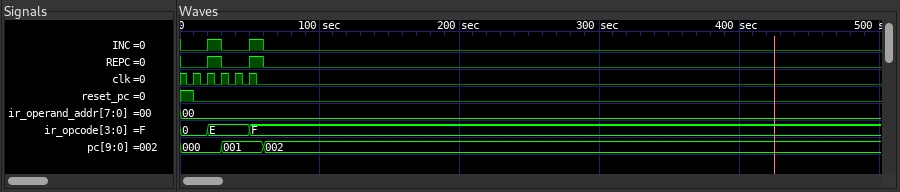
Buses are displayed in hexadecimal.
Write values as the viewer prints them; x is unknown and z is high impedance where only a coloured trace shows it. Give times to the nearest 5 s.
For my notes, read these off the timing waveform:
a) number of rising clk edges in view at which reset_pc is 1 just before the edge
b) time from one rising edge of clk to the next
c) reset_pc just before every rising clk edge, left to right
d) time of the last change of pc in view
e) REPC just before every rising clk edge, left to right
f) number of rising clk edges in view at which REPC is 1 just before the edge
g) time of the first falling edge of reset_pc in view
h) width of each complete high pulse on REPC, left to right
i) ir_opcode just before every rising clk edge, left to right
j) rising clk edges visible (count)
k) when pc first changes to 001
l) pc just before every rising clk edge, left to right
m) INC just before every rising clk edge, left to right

1
10 s
1 0 0 0 0
60 s
0 0 1 0 0
1
10 s
10 s, 10 s
0, 0, E, E, E
5
30 s
000, 000, 000, 001, 001
0 0 1 0 0
